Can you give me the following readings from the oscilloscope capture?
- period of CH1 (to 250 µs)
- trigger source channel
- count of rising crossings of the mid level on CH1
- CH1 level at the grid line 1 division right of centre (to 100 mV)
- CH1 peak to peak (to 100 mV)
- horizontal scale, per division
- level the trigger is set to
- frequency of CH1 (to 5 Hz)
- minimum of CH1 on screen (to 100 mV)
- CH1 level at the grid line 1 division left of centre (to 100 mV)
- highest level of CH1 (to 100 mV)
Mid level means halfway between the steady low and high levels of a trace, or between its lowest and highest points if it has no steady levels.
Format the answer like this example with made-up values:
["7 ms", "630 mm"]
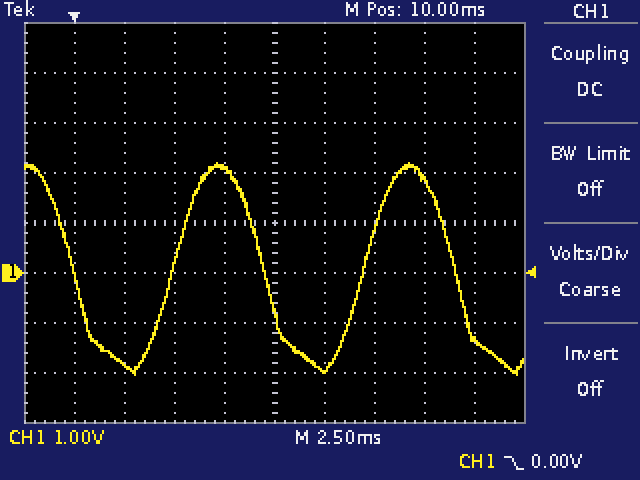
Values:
["9.50 ms", "CH1", "2", "-1.9 V", "4.2 V", "2.5 ms", "0.00 V", "105 Hz", "-2.0 V", "2.1 V", "2.2 V"]
